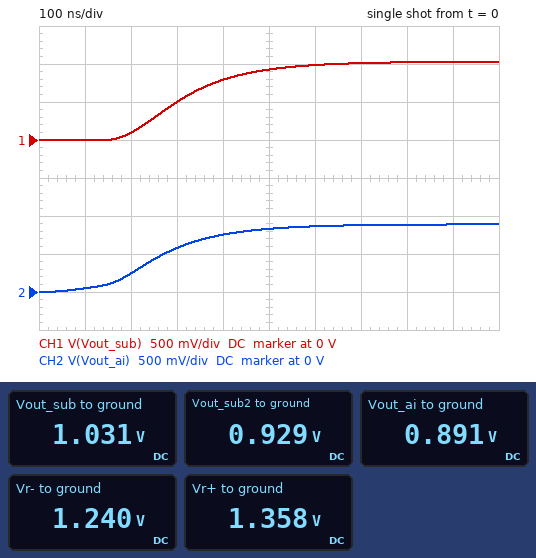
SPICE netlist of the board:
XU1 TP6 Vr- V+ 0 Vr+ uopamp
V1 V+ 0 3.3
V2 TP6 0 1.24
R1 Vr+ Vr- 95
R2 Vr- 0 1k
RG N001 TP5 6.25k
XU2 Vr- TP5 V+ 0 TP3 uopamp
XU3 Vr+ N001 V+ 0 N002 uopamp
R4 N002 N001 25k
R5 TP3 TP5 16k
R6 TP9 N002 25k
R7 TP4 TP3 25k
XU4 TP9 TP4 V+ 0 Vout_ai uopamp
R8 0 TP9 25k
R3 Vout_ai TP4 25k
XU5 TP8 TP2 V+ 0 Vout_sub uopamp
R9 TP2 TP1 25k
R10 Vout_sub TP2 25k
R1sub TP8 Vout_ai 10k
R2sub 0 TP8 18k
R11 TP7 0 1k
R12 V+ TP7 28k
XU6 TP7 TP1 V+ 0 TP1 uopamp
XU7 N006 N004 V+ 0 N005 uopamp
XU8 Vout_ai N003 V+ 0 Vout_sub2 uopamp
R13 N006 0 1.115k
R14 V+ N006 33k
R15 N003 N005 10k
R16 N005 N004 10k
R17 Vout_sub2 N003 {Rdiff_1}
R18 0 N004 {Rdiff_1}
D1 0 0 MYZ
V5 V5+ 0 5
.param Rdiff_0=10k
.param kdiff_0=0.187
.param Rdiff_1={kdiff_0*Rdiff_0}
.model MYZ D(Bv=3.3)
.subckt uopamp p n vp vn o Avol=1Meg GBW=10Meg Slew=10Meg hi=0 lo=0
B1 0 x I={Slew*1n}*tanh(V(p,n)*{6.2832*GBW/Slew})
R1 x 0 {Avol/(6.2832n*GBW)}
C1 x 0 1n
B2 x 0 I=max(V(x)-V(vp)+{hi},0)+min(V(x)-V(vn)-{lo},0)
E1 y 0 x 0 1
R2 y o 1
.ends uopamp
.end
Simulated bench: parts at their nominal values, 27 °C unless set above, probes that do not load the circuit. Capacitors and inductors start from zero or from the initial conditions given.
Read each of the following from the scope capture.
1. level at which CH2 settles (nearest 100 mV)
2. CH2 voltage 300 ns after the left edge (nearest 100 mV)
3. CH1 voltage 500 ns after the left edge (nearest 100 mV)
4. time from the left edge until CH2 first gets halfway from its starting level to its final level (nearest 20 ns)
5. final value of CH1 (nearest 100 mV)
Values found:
900 mV
600 mV
900 mV
260 ns
1.0 V
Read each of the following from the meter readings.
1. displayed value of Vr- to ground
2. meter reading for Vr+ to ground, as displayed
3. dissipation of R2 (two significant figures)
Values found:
1.240 V
1.358 V
1.5 mW
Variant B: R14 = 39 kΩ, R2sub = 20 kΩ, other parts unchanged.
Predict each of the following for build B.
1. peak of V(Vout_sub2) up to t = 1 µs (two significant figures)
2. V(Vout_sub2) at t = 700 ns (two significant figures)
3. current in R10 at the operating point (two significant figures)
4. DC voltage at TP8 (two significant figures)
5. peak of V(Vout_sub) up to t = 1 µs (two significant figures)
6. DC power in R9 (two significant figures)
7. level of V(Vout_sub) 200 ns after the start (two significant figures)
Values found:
950 mV
930 mV
19 µA
590 mV
1.1 V
9.2 µW
100 mV
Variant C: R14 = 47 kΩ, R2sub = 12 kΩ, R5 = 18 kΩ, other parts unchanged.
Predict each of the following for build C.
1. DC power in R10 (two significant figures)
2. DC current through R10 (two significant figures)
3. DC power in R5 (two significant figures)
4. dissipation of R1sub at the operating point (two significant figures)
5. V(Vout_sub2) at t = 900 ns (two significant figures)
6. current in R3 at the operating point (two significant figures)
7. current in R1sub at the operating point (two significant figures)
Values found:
6.2 µW
16 µA
6.4 µW
18 µW
1.0 V
550 nA
42 µA
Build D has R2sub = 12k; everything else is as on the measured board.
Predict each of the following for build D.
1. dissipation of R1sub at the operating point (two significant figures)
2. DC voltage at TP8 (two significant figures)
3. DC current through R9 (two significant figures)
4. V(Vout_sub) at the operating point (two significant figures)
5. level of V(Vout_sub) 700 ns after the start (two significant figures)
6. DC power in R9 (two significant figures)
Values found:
16 µW
490 mV
15 µA
860 mV
840 mV
5.5 µW
